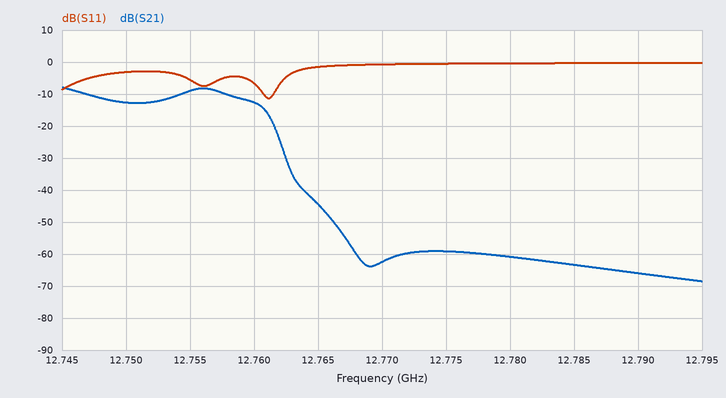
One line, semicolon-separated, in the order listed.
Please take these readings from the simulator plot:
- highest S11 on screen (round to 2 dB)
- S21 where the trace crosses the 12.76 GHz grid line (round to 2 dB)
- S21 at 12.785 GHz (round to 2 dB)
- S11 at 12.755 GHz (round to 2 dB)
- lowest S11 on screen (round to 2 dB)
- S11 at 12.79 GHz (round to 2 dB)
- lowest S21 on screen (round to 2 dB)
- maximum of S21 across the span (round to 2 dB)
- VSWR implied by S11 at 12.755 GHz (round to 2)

0 dB; -12 dB; -64 dB; -6 dB; -12 dB; 0 dB; -68 dB; -8 dB; 4
